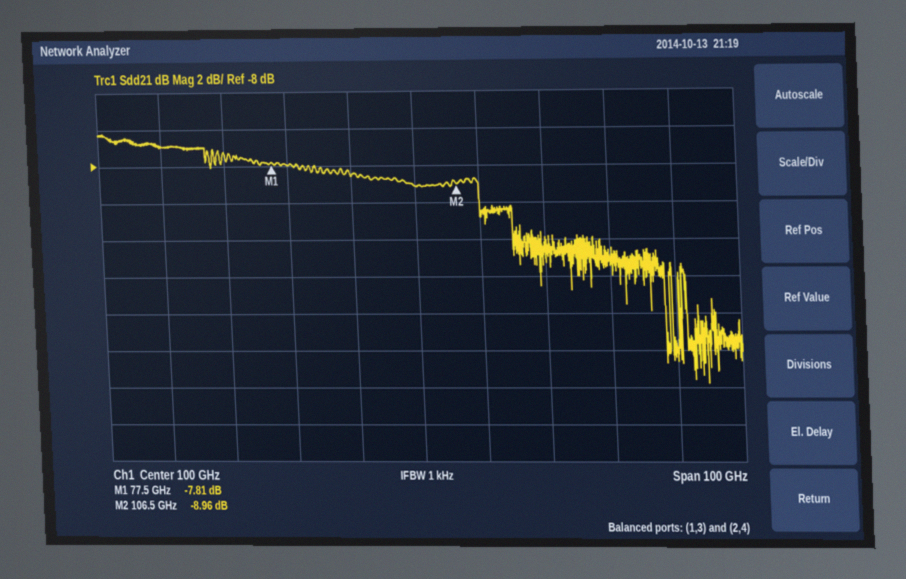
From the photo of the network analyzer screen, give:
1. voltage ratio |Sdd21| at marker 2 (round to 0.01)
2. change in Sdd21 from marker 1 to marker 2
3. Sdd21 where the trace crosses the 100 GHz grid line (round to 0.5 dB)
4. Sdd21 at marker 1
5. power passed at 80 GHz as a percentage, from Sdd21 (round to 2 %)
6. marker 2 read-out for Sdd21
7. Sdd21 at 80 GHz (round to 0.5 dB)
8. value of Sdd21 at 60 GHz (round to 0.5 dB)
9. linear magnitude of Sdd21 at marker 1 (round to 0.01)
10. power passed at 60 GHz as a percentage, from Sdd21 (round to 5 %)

0.36
-1.15 dB
-9.0 dB
-7.81 dB
16 %
-8.96 dB
-8.0 dB
-7.0 dB
0.41
20 %
